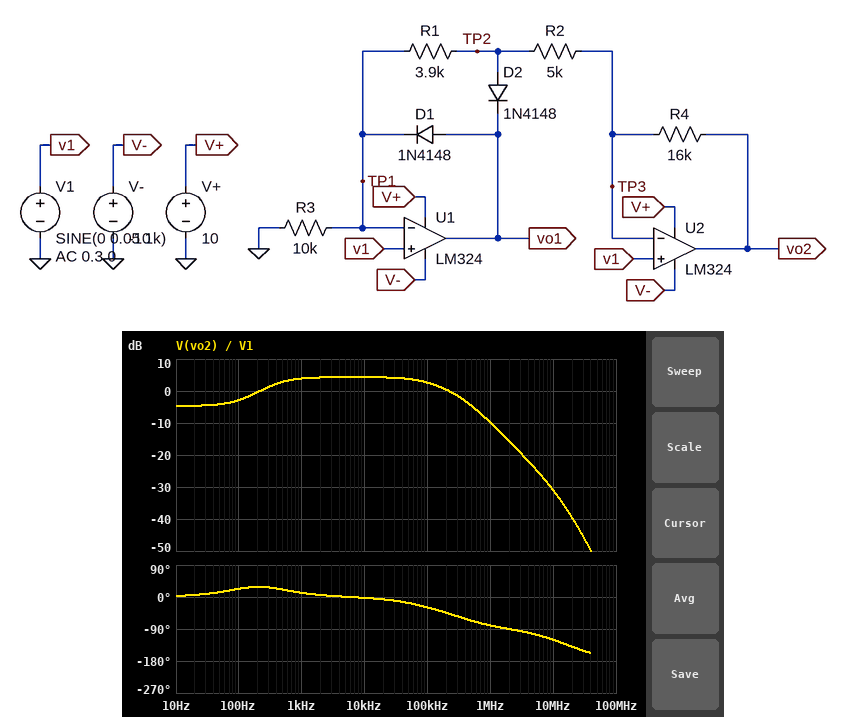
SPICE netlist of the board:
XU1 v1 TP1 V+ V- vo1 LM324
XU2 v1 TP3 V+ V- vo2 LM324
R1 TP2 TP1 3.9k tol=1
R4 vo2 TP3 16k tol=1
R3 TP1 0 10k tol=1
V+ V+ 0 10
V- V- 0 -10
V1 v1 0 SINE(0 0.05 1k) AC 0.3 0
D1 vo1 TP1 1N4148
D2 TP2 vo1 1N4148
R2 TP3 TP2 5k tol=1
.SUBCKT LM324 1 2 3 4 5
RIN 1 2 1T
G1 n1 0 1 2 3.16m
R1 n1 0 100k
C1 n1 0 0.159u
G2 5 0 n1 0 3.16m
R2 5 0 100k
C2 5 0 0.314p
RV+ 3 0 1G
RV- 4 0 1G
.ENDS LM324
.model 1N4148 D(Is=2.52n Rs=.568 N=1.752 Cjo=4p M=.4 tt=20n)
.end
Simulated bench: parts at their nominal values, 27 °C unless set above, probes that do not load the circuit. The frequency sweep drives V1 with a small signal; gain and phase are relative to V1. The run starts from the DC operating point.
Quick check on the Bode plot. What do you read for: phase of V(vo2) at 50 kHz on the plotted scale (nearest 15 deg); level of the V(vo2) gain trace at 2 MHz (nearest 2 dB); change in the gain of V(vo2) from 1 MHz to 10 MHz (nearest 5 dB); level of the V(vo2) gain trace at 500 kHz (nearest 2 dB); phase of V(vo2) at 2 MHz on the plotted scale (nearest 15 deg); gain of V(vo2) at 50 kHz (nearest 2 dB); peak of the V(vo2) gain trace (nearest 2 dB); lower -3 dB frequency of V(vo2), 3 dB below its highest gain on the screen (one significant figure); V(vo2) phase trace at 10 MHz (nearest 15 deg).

-15 deg
-16 dB
-20 dB
-4 dB
-90 deg
4 dB
4 dB
300 Hz
-120 deg
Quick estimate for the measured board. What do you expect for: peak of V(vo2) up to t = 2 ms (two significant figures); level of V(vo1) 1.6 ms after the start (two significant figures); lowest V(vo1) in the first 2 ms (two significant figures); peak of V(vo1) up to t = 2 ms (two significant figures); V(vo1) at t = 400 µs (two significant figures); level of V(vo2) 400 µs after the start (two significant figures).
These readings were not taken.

50 mV
-380 mV
-440 mV
390 mV
350 mV
29 mV
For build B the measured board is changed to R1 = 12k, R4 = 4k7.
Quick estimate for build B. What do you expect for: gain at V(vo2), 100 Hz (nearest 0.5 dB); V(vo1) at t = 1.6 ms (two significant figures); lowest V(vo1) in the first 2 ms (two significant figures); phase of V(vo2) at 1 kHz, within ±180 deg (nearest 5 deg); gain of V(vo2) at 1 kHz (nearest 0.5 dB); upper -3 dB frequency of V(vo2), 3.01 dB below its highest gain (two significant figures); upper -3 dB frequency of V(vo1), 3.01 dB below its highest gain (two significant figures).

-2.0 dB
-430 mV
-510 mV
5 deg
0.5 dB
310 kHz
380 Hz
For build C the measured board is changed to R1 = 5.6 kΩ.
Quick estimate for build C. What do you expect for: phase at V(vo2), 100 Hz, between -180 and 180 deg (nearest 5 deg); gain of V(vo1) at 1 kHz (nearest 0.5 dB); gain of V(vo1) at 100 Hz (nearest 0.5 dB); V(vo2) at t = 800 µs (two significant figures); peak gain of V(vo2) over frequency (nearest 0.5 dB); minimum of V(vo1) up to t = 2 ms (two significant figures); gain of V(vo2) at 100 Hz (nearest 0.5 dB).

30 deg
52.0 dB
61.0 dB
40 mV
4.0 dB
-460 mV
-4.5 dB
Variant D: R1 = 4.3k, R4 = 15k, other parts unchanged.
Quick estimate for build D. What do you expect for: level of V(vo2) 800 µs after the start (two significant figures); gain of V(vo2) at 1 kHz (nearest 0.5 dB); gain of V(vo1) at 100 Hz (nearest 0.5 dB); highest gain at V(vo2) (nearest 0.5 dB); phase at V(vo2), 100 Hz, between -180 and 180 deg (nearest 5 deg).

15 mV
3.5 dB
61.0 dB
4.0 dB
20 deg
